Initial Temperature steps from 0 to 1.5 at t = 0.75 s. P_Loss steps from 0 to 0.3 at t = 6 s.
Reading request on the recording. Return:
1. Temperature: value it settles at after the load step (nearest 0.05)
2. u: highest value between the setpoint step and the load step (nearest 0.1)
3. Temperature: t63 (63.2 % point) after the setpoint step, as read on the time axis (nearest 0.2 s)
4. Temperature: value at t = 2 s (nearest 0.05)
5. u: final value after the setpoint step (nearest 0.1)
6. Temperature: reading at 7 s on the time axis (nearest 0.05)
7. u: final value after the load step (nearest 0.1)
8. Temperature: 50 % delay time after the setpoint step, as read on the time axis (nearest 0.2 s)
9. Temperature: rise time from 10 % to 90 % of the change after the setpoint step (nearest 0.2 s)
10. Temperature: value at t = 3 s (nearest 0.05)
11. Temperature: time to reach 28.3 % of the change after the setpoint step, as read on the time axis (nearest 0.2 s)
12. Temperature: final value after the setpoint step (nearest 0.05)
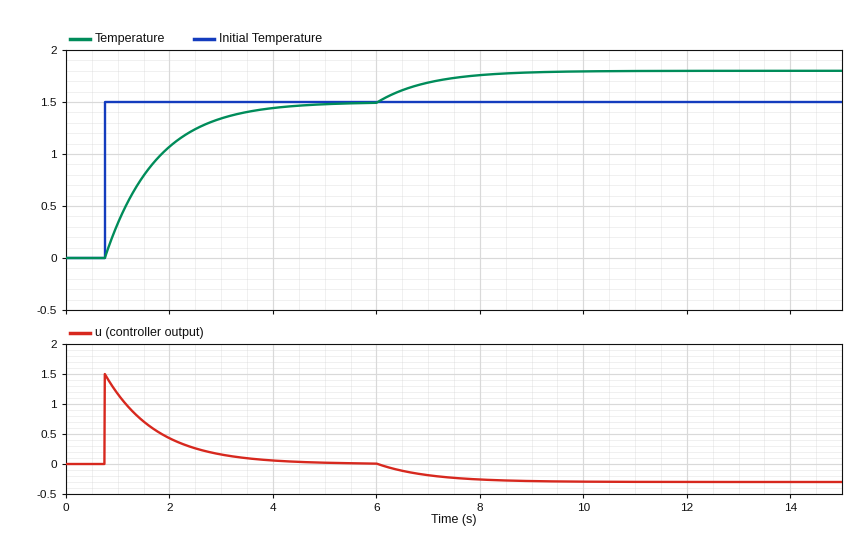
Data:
1.80
1.5
1.8 s
1.05
0.0
1.70
-0.3
1.4 s
2.2 s
1.35
1.0 s
1.50
